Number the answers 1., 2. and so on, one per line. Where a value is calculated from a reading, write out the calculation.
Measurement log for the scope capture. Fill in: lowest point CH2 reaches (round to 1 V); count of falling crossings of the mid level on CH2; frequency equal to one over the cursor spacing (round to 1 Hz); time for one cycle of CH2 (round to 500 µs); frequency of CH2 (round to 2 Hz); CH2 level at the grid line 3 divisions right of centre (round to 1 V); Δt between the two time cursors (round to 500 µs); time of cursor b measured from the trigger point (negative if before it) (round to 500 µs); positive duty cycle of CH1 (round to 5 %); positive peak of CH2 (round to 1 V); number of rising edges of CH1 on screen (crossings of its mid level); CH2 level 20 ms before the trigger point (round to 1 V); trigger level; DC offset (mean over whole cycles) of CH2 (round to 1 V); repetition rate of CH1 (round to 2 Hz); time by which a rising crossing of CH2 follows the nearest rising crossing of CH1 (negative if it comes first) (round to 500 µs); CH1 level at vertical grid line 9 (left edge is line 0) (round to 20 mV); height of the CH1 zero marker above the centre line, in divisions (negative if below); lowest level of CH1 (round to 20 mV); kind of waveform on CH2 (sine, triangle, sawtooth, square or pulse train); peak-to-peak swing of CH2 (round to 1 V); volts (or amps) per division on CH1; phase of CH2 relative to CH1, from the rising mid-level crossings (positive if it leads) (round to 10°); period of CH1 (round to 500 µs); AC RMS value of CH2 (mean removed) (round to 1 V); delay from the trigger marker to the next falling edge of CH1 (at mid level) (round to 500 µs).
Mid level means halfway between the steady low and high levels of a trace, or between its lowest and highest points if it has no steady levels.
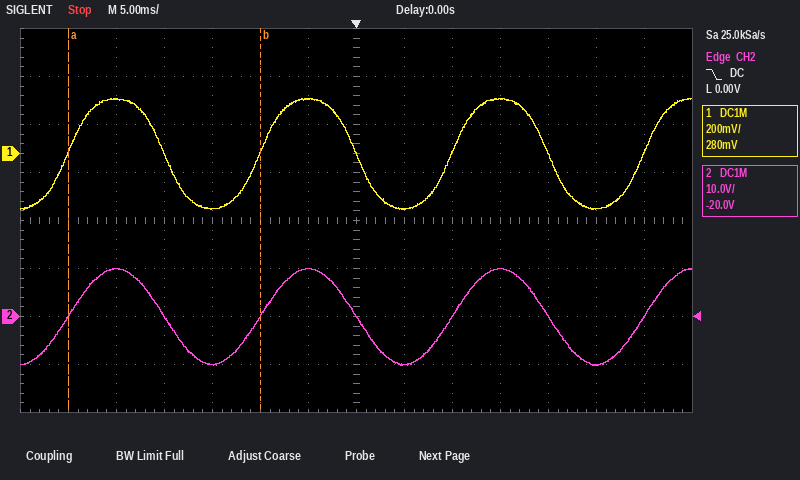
1. -10 V
2. 3
3. 1 / 20.0 ms ≈ 50 Hz
4. 20.0 ms
5. 1 / 20.0 ms ≈ 50 Hz
6. 10 V
7. 20.0 ms
8. -10.0 ms
9. 50 %
10. 10 V
11. 4
12. 0 V
13. 0.00 V
14. (10 V + (-10 V)) / 2 ≈ 0 V
15. 1 / 20.0 ms ≈ 50 Hz
16. 0.0 ms
17. 0 mV
18. +1.4 div
19. -240 mV
20. sine
21. 10 V − (-10 V) = 20 V
22. 200 mV
23. −360° × (0.0 ms) / 20.0 ms ≈ 0°
24. 20.0 ms
25. 20 V / (2√2) ≈ 7 V
26. 20.0 ms
